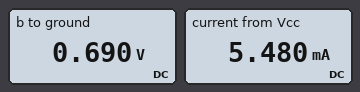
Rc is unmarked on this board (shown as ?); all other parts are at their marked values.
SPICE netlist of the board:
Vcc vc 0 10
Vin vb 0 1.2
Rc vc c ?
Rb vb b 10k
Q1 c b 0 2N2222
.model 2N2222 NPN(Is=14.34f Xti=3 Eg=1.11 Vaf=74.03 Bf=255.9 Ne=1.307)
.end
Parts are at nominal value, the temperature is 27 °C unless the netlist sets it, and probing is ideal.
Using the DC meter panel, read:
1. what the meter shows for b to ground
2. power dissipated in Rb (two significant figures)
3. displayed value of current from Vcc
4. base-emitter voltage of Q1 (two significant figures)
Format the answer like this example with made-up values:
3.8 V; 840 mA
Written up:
0.690 V; 26 µW; 5.480 mA; 690 mV
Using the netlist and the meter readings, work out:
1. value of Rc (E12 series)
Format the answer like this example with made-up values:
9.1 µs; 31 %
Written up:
1.8 kΩ
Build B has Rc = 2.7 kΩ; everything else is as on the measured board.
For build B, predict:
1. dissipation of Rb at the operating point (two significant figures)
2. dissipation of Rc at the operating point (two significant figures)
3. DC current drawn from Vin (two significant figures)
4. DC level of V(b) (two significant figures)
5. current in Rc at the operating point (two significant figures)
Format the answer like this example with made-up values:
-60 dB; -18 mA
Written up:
27 µW; 36 mW; 52 µA; 680 mV; 3.7 mA
